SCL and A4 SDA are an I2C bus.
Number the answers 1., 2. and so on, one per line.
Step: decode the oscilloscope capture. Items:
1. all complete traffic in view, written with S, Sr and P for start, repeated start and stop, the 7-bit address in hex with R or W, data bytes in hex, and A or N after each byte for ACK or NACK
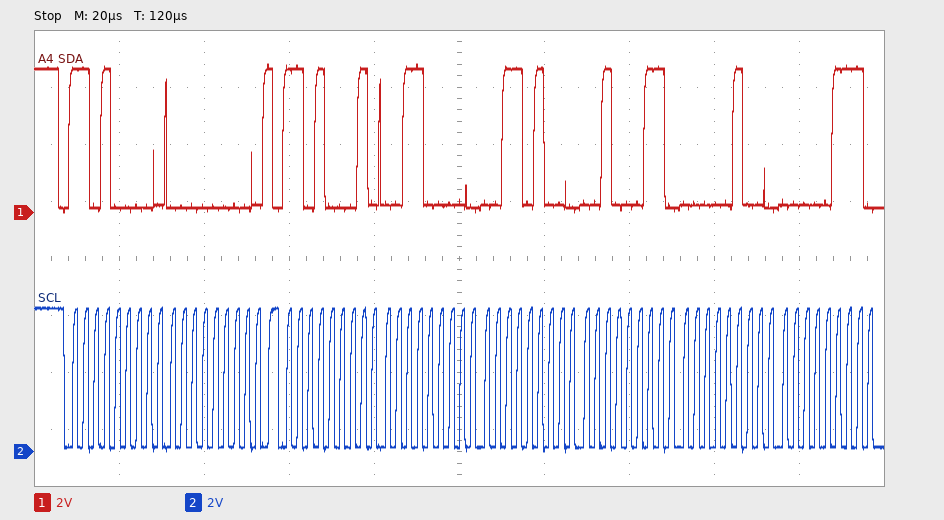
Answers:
1. S 68W A 00 A Sr 68R A 30 A 34 A 23 A 04 A 07 A
